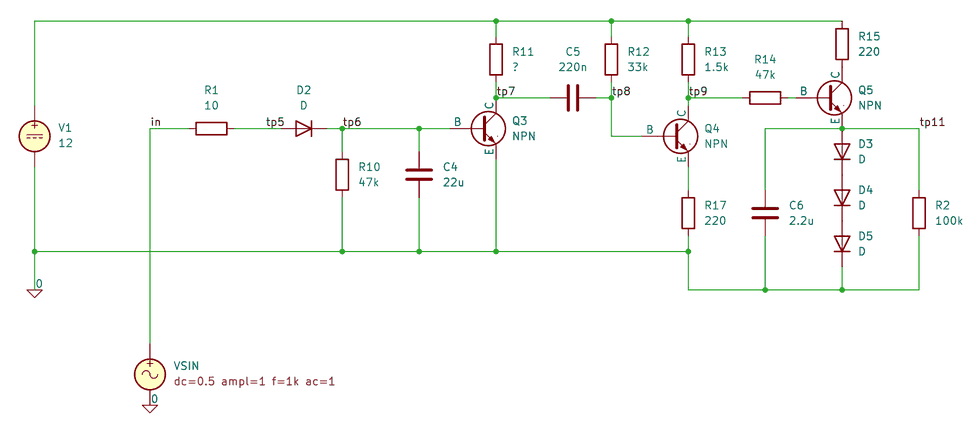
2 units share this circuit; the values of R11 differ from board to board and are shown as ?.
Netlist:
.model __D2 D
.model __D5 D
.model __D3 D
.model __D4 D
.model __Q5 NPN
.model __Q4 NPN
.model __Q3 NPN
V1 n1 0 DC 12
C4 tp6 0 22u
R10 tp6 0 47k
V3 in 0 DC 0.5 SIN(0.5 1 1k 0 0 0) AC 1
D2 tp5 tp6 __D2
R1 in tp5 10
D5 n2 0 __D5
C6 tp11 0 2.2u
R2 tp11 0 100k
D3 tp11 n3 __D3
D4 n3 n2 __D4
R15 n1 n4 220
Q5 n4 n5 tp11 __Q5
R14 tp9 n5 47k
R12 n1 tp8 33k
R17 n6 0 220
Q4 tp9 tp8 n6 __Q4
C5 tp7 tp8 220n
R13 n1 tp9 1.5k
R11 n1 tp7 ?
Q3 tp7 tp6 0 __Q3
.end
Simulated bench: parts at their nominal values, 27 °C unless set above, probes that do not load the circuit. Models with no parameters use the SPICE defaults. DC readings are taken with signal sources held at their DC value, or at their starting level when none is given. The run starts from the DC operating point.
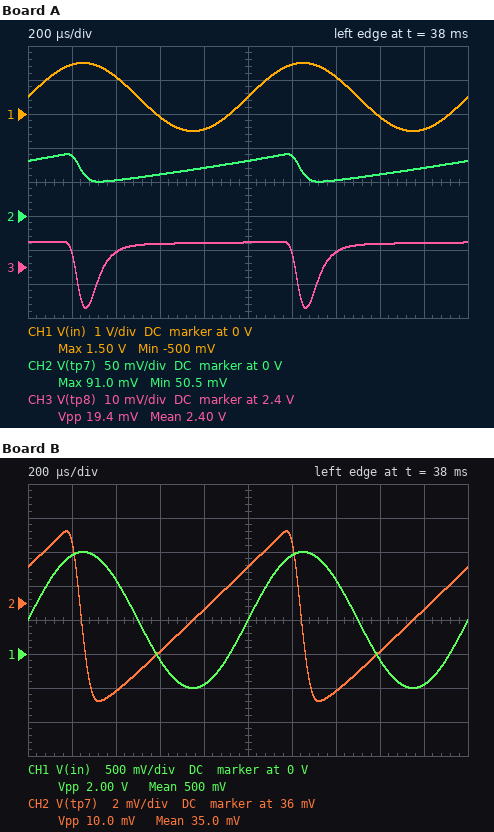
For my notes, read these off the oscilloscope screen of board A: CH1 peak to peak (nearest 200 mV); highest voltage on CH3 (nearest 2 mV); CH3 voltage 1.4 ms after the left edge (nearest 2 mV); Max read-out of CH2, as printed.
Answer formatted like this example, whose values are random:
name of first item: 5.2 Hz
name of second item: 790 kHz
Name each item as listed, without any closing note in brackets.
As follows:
CH1 peak to peak: 2.0 V
highest voltage on CH3: 2.408 V
CH3 voltage 1.4 ms after the left edge: 2.404 V
Max read-out of CH2, as printed: 91.0 mV
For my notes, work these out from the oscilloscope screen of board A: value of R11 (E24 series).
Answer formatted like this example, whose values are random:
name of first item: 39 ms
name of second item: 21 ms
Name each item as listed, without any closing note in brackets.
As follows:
value of R11: 6.8 kΩ
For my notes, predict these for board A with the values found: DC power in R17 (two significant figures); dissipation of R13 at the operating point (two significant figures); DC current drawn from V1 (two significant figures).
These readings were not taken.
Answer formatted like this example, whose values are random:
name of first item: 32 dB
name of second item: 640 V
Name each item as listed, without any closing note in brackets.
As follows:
DC power in R17: 11 mW
dissipation of R13 at the operating point: 71 mW
DC current drawn from V1: 7.2 mA
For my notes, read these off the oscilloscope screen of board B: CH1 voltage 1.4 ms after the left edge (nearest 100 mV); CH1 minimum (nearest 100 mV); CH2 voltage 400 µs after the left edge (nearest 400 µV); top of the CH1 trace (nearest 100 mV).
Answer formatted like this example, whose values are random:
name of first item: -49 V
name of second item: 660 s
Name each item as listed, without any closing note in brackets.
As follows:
CH1 voltage 1.4 ms after the left edge: 1.1 V
CH1 minimum: -500 mV
CH2 voltage 400 µs after the left edge: 30.8 mV
top of the CH1 trace: 1.5 V
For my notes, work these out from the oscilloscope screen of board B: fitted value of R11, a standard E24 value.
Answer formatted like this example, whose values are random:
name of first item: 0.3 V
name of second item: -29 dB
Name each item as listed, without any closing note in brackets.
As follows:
fitted value of R11, a standard E24 value: 24 kΩ
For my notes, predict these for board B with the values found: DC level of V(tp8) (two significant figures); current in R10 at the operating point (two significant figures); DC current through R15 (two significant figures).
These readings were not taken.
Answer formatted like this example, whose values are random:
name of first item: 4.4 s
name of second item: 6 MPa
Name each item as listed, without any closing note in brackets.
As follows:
DC level of V(tp8): 2.4 V
current in R10 at the operating point: 700 nA
DC current through R15: 10 µA
